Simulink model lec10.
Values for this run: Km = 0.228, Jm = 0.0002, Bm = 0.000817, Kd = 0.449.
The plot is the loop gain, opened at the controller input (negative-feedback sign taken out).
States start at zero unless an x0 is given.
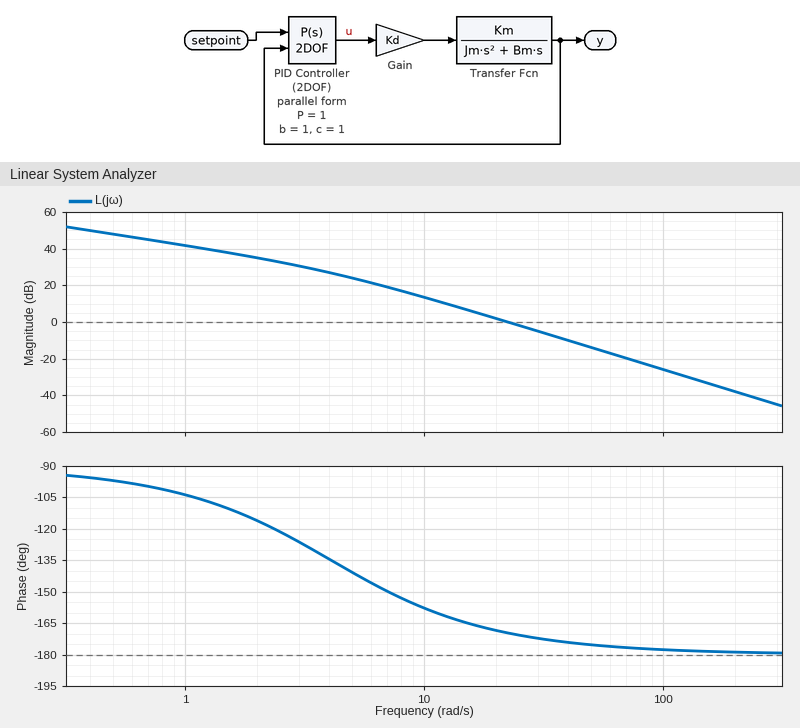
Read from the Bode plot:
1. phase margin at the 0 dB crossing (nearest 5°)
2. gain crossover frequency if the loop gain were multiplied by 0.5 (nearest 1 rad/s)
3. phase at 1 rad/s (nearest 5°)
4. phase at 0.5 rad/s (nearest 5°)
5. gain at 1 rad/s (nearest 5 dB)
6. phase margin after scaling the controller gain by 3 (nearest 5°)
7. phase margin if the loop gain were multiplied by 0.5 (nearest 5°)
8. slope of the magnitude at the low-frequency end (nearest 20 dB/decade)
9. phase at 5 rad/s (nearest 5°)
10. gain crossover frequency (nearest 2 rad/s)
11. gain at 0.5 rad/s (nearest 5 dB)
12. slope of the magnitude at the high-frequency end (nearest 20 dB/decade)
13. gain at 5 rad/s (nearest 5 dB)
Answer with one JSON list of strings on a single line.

["10°", "16 rad/s", "-105°", "-95°", "40 dB", "5°", "15°", "-20 dB/decade", "-140°", "22 rad/s", "50 dB", "-40 dB/decade", "25 dB"]
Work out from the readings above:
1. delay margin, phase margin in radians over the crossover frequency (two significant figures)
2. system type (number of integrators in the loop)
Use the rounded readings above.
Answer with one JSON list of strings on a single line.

["0.0079 s", "1"]
